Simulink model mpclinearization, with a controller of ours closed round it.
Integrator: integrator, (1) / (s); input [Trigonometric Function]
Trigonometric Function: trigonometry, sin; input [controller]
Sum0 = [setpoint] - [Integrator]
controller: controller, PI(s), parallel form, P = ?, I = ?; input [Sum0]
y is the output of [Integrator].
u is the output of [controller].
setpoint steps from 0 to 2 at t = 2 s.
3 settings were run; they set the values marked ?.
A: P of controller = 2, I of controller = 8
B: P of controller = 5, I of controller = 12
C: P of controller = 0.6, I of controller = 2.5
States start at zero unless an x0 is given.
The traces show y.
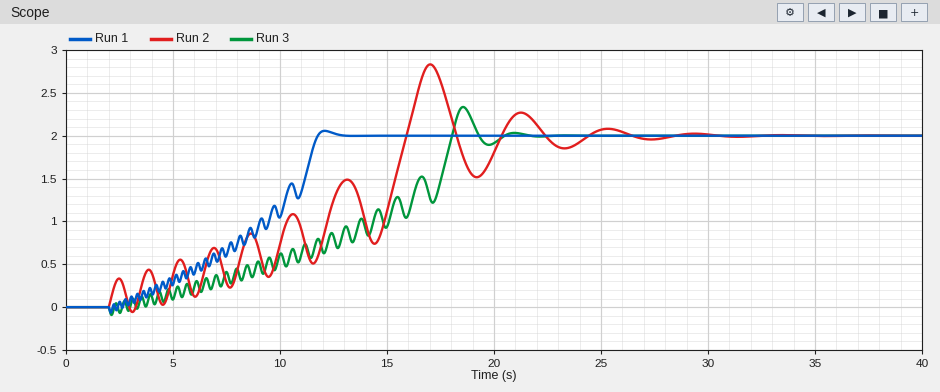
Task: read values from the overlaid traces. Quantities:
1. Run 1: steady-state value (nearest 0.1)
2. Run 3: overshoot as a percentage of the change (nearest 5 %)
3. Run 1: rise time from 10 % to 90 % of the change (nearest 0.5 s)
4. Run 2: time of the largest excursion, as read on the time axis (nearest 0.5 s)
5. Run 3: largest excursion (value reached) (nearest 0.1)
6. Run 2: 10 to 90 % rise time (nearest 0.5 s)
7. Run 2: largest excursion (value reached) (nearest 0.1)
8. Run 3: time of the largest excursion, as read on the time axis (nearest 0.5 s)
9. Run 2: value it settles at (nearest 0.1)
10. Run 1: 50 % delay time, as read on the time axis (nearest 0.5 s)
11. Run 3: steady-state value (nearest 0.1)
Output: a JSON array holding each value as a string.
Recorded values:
["2.0", "15 %", "7.5 s", "17.0 s", "2.3", "13.5 s", "2.8", "18.5 s", "2.0", "9.0 s", "2.0"]
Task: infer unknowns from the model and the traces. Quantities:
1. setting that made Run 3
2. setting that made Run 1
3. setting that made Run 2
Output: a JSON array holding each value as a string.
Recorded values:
["A", "B", "C"]
